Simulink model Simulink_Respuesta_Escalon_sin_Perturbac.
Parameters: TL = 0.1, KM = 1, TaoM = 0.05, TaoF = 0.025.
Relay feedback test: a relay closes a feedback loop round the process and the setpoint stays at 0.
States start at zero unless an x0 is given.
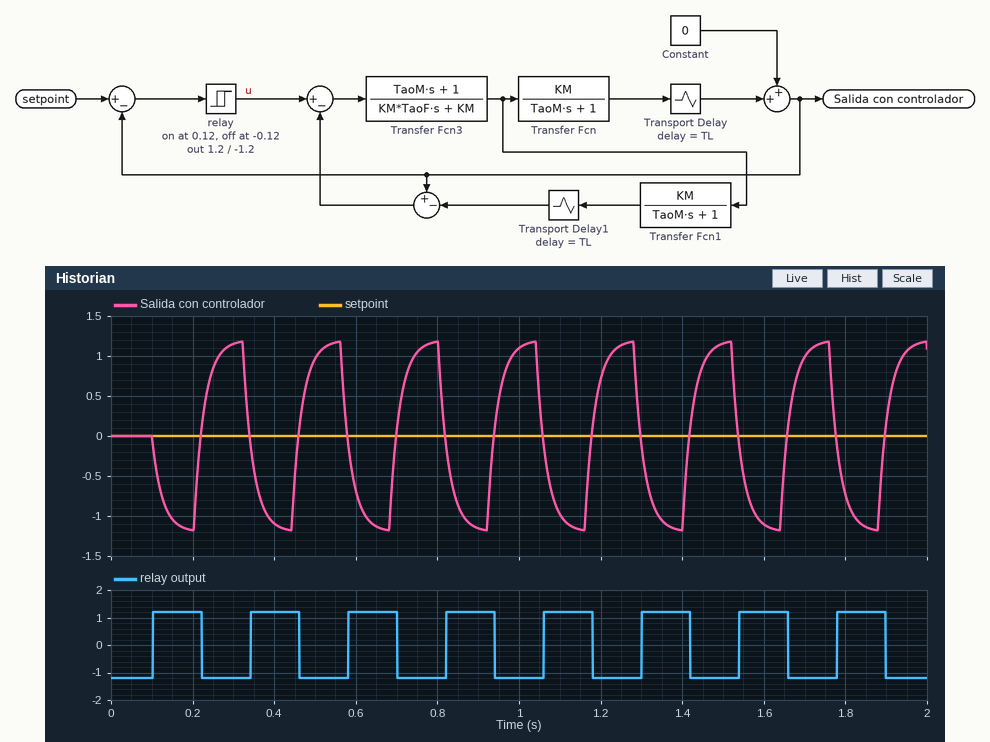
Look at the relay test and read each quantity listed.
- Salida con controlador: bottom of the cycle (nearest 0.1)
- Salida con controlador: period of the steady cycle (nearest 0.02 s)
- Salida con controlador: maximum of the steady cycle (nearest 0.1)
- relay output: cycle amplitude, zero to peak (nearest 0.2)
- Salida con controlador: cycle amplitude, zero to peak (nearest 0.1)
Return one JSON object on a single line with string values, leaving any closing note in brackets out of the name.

{"Salida con controlador: bottom of the cycle": "-1.2", "Salida con controlador: period of the steady cycle": "0.24 s", "Salida con controlador: maximum of the steady cycle": "1.2", "relay output: cycle amplitude, zero to peak": "1.2", "Salida con controlador: cycle amplitude, zero to peak": "1.2"}
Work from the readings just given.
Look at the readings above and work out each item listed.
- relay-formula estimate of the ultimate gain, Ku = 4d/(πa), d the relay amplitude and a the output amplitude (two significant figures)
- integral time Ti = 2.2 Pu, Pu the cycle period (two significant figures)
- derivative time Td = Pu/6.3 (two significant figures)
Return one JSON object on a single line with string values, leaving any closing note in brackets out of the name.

{"relay-formula estimate of the ultimate gain, Ku = 4d/(πa), d the relay amplitude and a the output amplitude": "1.3", "integral time Ti = 2.2 Pu, Pu the cycle period": "0.53 s", "derivative time Td = Pu/6.3": "0.038 s"}
